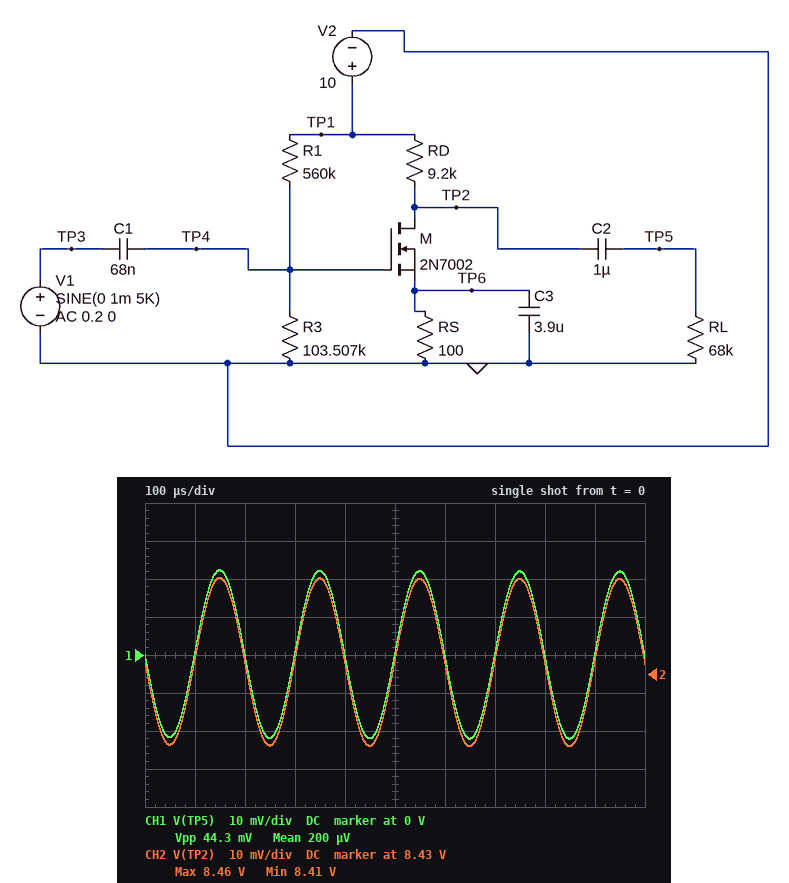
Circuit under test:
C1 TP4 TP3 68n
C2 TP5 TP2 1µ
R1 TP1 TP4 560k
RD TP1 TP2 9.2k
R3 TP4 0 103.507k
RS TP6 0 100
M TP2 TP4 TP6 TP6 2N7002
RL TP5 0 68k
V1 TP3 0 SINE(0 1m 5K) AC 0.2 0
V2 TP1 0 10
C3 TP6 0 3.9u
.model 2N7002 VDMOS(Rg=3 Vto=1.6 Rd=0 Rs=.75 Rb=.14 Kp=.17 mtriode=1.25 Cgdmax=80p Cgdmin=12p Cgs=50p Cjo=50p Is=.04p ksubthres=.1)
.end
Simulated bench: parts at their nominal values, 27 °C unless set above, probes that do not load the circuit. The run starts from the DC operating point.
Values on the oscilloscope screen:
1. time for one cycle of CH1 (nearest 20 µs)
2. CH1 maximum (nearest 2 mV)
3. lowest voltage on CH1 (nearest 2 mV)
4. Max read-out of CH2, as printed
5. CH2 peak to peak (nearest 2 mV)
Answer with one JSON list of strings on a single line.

["200 µs", "22 mV", "-22 mV", "8.46 V", "44 mV"]
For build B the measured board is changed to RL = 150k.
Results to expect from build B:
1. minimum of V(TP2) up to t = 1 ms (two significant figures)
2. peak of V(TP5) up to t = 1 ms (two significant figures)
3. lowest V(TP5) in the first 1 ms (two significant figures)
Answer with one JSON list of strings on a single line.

["8.4 V", "24 mV", "-24 mV"]
